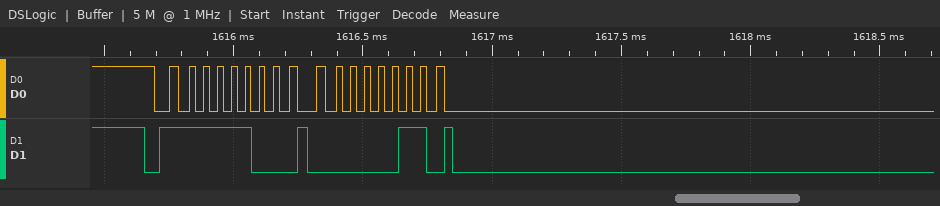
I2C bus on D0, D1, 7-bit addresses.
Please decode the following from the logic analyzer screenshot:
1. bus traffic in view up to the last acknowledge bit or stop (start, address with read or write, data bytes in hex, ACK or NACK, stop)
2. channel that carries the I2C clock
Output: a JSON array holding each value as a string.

["start, address 7E write ACK, 03 ACK", "D0"]
